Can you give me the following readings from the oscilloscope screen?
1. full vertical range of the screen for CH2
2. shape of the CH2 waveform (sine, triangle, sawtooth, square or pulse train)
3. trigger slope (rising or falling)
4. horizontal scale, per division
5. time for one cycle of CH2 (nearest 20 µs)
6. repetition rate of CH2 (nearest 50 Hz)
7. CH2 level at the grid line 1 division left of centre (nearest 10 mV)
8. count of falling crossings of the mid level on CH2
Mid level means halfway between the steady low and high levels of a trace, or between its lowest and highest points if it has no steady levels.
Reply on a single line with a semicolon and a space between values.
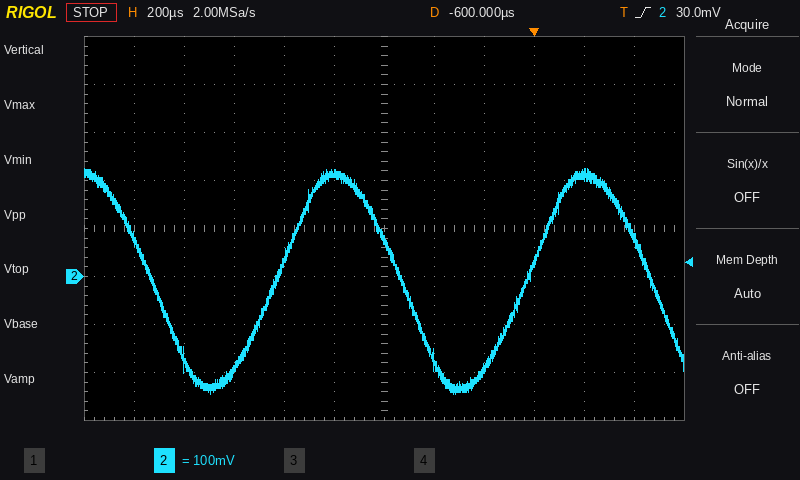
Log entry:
800 mV; sine; rising; 200 µs; 1.00 ms; 1.00 kHz; 210 mV; 3
